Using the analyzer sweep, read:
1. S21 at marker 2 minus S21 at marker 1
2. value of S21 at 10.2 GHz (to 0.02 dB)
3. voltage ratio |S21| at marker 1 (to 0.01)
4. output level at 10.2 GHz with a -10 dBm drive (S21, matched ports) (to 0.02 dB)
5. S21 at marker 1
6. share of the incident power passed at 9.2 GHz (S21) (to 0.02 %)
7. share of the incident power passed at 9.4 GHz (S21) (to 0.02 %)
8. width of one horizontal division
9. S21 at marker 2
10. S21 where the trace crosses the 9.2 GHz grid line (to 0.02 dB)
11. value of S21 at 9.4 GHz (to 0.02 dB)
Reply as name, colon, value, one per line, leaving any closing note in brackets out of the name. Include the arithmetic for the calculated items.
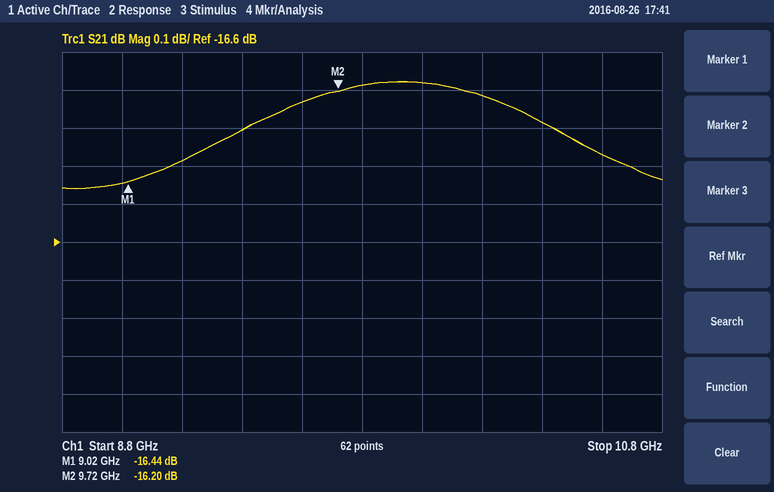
S21 at marker 2 minus S21 at marker 1: -16.2 − (-16.44) = 0.24 dB
value of S21 at 10.2 GHz: -16.22 dB
voltage ratio |S21| at marker 1: 10^(-16.44/20) ≈ 0.15
output level at 10.2 GHz with a -10 dBm drive (S21, matched ports): -10 dBm + (-16.22 dB) = -26.22 dBm
S21 at marker 1: -16.44 dB
share of the incident power passed at 9.2 GHz (S21): 10^(-16.38/10) ≈ 2.30 %
share of the incident power passed at 9.4 GHz (S21): 10^(-16.3/10) ≈ 2.34 %
width of one horizontal division: 200 MHz
S21 at marker 2: -16.20 dB
S21 where the trace crosses the 9.2 GHz grid line: -16.38 dB
value of S21 at 9.4 GHz: -16.30 dB
